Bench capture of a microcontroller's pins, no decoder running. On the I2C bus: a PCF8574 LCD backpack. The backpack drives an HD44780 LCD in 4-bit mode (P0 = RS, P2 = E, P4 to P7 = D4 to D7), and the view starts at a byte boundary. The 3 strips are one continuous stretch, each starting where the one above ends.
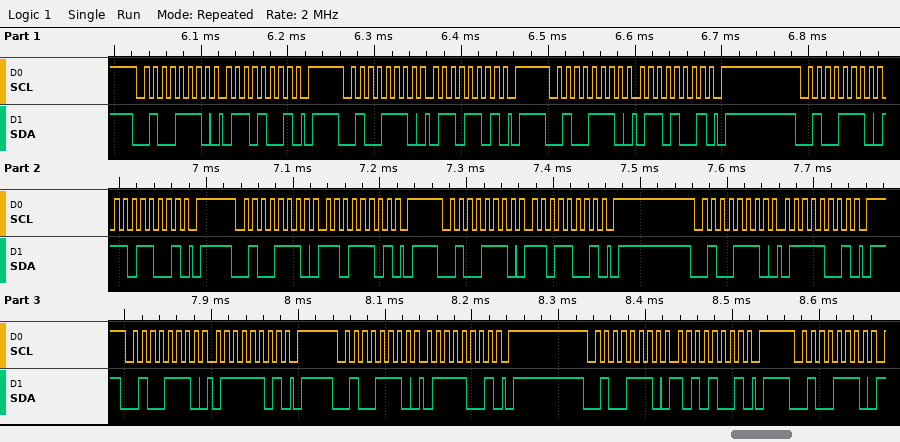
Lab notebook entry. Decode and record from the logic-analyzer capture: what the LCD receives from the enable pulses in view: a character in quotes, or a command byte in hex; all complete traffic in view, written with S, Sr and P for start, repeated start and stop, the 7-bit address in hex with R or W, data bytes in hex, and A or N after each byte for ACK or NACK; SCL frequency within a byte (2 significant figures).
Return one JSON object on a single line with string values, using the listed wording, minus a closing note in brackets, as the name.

{"what the LCD receives from the enable pulses in view: a character in quotes, or a command byte in hex": "'m'", "all complete traffic in view, written with S, Sr and P for start, repeated start and stop, the 7-bit address in hex with R or W, data bytes in hex, and A or N after each byte for ACK or NACK": "S 27W A 69 A P S 27W A 6D A P S 27W A 69 A P S 27W A D9 A P S 27W A DD A P S 27W A D9 A P S 27W A 79 A P S 27W A 7D A P S 27W A 79 A P S 27W A A9 A P S 27W A", "SCL frequency within a byte": "100 kHz"}
